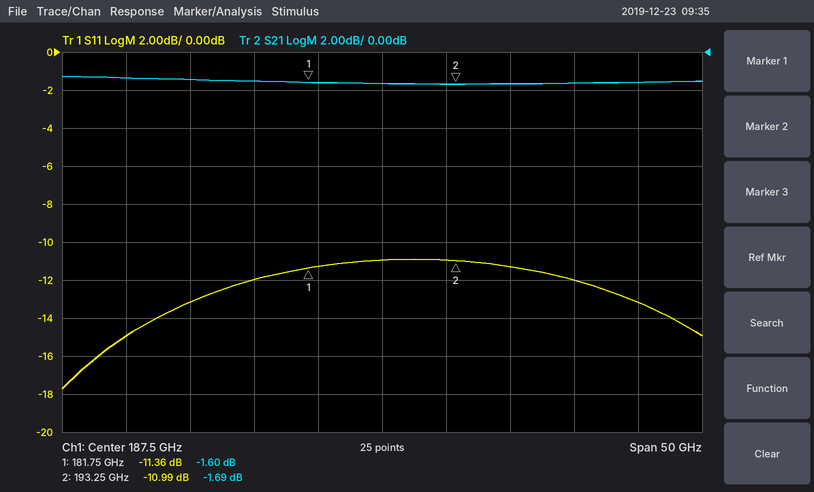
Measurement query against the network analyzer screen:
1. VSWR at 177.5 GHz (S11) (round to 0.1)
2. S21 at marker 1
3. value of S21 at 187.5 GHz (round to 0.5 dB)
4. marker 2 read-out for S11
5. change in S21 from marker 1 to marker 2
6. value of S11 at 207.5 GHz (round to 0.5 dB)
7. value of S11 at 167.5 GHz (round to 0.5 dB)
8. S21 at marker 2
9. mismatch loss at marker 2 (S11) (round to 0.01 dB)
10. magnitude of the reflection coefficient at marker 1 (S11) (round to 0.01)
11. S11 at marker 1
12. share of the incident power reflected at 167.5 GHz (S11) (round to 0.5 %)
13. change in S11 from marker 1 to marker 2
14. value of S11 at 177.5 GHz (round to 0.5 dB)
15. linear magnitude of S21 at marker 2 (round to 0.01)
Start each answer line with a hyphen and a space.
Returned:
- 1.7
- -1.60 dB
- -1.5 dB
- -10.99 dB
- -0.09 dB
- -13.0 dB
- -15.0 dB
- -1.69 dB
- 0.36 dB
- 0.27
- -11.36 dB
- 3.0 %
- 0.37 dB
- -12.0 dB
- 0.82
